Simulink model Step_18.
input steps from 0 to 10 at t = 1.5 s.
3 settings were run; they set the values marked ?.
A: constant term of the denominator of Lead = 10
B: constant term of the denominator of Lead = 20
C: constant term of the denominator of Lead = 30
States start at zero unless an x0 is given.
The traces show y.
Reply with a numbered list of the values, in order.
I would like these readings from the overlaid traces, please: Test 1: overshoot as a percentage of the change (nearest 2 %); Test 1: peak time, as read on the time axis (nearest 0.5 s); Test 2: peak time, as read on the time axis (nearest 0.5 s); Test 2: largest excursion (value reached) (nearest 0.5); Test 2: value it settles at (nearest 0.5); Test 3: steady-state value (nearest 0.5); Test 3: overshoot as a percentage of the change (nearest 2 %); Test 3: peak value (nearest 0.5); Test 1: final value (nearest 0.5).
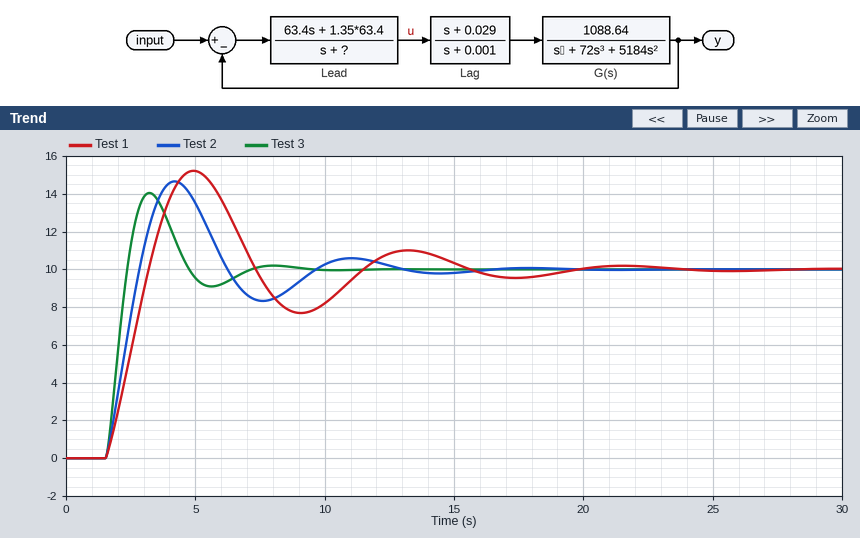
1. 52 %
2. 5.0 s
3. 4.0 s
4. 14.5
5. 10.0
6. 10.0
7. 40 %
8. 14.0
9. 10.0
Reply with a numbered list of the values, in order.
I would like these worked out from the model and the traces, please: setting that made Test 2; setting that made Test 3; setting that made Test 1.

1. B
2. A
3. C
